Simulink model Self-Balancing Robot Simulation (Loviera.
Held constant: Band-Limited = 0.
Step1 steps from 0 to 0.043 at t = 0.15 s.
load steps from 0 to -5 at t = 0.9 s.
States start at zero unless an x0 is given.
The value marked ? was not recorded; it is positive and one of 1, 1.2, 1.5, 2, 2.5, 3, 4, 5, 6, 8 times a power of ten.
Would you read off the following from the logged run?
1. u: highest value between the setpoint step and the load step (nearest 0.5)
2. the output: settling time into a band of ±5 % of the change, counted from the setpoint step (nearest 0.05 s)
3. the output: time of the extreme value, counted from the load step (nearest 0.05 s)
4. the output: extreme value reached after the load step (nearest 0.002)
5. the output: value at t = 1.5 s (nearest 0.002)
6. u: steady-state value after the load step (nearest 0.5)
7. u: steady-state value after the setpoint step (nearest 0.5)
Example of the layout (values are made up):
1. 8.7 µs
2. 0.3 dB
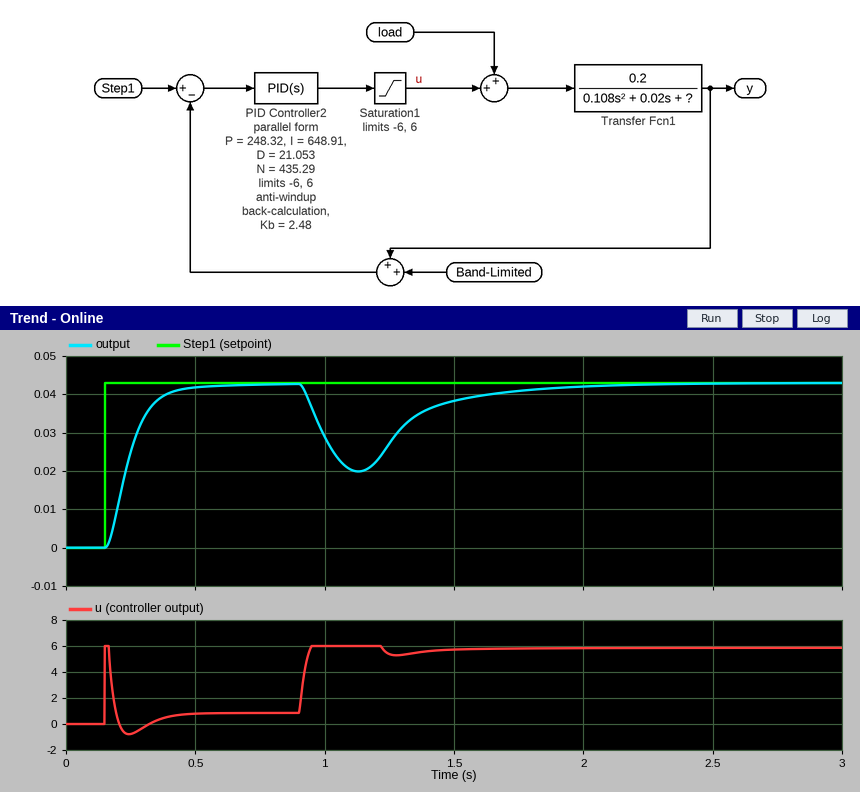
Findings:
1. 6.0
2. 0.25 s
3. 0.25 s
4. 0.020
5. 0.038
6. 6.0
7. 1.0
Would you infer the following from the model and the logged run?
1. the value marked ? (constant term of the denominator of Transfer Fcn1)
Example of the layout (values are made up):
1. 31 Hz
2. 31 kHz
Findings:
1. 4
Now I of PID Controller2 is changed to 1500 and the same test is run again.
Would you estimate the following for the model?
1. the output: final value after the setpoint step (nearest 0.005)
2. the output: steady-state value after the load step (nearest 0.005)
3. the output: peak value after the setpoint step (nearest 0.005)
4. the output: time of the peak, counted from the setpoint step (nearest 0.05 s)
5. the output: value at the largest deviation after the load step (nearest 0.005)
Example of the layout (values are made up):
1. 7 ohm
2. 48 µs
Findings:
1. 0.045
2. 0.045
3. 0.050
4. 0.25 s
5. 0.020
